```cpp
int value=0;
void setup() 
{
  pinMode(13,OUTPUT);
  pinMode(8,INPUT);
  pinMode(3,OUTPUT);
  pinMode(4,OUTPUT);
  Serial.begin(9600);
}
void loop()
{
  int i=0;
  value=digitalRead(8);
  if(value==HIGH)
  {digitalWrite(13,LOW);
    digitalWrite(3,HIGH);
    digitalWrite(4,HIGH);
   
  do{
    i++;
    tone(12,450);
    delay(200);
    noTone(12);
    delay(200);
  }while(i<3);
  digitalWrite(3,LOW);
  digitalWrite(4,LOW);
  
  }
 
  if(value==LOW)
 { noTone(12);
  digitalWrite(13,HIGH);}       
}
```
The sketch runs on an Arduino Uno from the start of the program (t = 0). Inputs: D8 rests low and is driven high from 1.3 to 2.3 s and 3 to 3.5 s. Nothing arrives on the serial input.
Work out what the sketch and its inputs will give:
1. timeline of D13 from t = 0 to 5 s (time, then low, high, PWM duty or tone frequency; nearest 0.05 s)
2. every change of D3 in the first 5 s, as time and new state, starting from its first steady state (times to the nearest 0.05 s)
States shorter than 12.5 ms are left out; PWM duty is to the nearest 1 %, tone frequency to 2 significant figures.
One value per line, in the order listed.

0 s high; 1.3 s low; 2.5 s high; 3 s low; 4.2 s high
0 s low; 1.3 s high; 2.5 s low; 3 s high; 4.2 s low
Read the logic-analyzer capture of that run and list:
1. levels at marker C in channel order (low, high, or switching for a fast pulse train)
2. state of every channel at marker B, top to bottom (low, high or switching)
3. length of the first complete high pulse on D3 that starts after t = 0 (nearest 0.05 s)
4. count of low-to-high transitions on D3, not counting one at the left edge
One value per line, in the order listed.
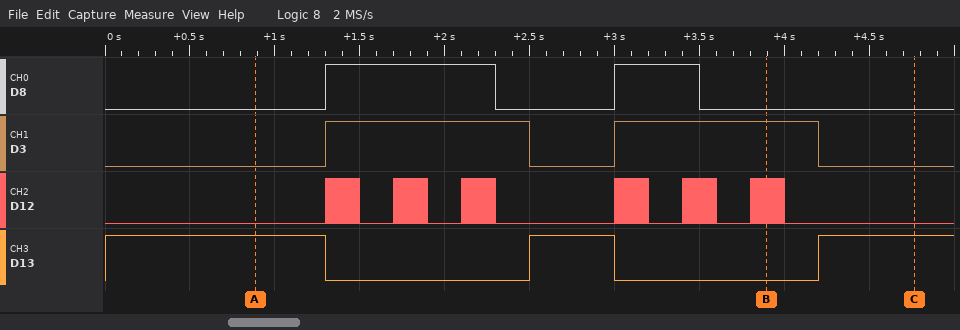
D8 low, D3 low, D12 low, D13 high
D8 low, D3 high, D12 switching, D13 low
1.20 s
2
